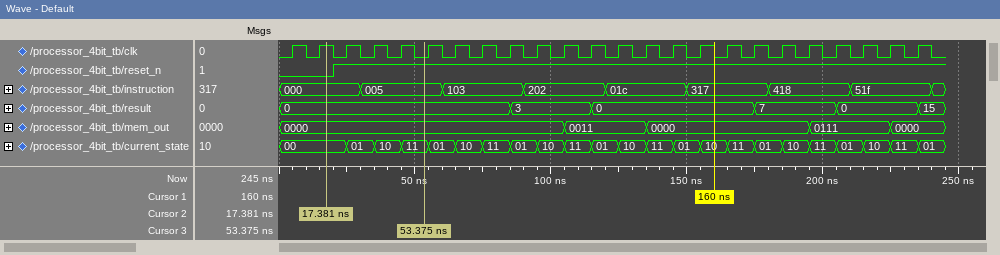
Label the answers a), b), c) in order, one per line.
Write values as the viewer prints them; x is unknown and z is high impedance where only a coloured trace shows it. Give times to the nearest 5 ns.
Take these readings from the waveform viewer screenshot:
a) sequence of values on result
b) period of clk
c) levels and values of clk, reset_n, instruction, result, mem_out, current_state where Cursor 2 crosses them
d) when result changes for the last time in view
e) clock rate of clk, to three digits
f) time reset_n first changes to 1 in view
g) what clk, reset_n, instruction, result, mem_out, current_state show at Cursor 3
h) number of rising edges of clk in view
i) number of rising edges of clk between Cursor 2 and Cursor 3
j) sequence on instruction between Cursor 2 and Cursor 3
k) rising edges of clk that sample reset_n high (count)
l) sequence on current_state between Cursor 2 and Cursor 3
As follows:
a) 0, 3, 0, 7, 0, 15
b) 10 ns
c) clk=1, reset_n=0, instruction=000, result=0, mem_out=0000, current_state=00
d) 235 ns
e) 100 MHz
f) 20 ns
g) clk=0, reset_n=1, instruction=005, result=0, mem_out=0000, current_state=11
h) 24
i) 3
j) 000, 005
k) 22
l) 00, 01, 10, 11
